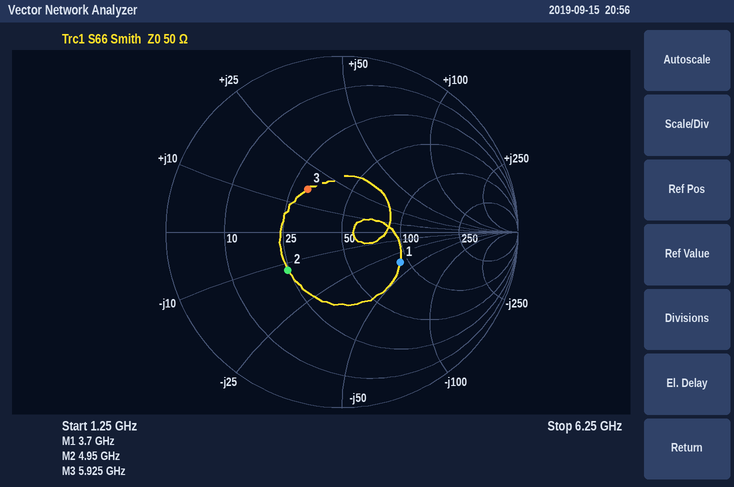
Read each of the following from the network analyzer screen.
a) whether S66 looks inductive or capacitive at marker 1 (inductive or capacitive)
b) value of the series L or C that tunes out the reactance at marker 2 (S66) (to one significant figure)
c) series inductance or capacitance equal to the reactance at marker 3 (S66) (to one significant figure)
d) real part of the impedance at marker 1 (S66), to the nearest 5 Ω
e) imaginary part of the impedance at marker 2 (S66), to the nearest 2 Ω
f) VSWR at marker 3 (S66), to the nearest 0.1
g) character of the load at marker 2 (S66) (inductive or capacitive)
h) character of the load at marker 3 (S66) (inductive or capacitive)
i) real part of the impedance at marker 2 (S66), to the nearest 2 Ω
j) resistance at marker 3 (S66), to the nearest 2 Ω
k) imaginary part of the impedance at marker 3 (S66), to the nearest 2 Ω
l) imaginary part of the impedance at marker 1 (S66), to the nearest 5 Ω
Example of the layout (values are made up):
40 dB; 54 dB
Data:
capacitive; 400 pH; 400 pH; 90 Ω; -12 Ω; 1.9; capacitive; inductive; 24 Ω; 30 Ω; +16 Ω; -35 Ω
